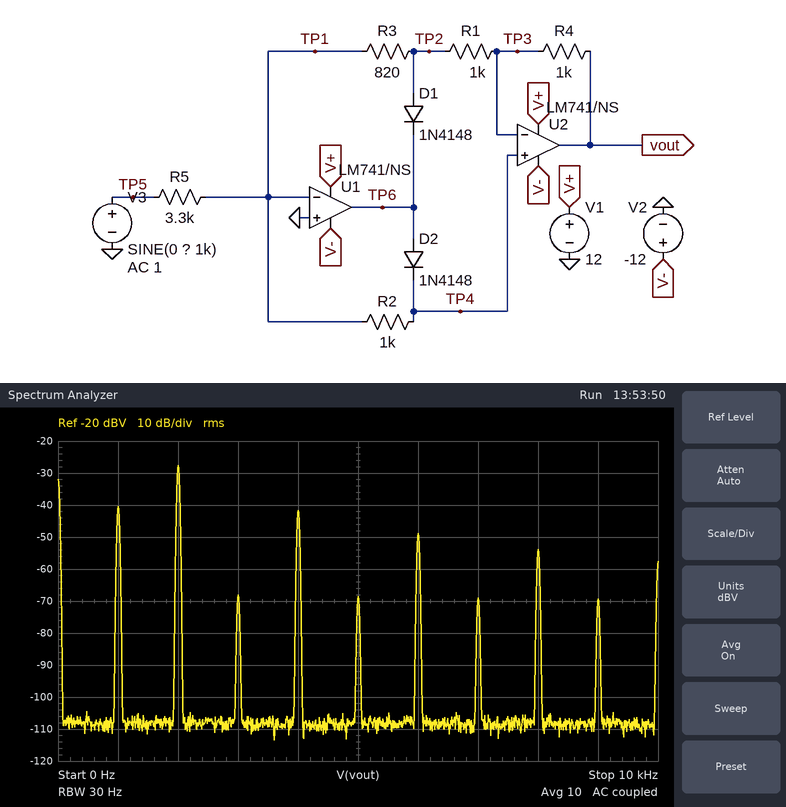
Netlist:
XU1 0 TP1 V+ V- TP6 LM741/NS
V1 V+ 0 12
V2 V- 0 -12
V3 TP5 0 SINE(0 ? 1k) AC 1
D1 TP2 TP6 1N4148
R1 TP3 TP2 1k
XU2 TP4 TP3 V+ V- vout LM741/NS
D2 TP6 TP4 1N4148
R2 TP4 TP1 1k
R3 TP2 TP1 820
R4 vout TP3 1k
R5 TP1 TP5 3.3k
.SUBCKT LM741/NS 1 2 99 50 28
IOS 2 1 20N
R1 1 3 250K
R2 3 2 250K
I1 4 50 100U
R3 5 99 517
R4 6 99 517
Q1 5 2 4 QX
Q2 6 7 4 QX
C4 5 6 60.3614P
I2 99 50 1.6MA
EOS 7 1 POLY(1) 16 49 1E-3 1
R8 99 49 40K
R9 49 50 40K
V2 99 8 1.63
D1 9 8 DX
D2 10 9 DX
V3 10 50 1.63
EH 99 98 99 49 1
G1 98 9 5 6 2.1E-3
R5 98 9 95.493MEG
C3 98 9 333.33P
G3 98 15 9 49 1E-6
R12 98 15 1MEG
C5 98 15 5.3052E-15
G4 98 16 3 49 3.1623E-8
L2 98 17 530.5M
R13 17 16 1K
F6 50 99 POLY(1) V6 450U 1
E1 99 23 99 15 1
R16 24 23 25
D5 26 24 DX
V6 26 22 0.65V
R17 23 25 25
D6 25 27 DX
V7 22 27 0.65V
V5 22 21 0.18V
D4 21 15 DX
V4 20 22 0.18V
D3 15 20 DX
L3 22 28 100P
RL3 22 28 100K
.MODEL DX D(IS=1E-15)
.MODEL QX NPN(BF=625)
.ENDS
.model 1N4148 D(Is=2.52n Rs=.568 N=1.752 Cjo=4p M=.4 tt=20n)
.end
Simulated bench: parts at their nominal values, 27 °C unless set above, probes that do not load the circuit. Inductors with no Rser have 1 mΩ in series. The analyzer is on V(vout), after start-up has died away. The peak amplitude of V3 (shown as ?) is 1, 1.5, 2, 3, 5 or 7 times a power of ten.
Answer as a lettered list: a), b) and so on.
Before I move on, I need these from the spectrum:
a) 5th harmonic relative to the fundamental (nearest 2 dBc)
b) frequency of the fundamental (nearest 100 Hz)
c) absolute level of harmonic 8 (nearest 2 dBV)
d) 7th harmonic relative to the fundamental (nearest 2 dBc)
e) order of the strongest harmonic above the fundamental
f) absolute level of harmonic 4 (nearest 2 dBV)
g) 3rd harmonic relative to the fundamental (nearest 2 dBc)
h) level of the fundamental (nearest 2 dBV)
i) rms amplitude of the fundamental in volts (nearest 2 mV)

a) -28 dBc
b) 1.0 kHz
c) -54 dBV
d) -28 dBc
e) 2
f) -42 dBV
g) -28 dBc
h) -40 dBV
i) 10 mV
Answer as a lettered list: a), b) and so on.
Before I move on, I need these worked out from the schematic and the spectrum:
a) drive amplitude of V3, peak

a) 500 mV
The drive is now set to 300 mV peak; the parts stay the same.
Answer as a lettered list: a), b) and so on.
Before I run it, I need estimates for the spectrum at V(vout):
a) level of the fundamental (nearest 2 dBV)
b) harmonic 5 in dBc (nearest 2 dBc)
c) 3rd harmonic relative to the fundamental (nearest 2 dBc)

a) -44 dBV
b) -24 dBc
c) -24 dBc
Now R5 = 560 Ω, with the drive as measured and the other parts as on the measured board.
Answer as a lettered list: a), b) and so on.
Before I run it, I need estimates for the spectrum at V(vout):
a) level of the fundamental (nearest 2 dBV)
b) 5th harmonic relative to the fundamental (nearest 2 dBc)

a) -24 dBV
b) -40 dBc
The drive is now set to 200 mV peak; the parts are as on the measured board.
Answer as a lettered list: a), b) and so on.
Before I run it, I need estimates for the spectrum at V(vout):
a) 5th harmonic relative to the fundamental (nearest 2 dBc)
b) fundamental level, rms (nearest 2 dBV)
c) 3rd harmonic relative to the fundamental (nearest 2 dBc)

a) -22 dBc
b) -48 dBV
c) -20 dBc
